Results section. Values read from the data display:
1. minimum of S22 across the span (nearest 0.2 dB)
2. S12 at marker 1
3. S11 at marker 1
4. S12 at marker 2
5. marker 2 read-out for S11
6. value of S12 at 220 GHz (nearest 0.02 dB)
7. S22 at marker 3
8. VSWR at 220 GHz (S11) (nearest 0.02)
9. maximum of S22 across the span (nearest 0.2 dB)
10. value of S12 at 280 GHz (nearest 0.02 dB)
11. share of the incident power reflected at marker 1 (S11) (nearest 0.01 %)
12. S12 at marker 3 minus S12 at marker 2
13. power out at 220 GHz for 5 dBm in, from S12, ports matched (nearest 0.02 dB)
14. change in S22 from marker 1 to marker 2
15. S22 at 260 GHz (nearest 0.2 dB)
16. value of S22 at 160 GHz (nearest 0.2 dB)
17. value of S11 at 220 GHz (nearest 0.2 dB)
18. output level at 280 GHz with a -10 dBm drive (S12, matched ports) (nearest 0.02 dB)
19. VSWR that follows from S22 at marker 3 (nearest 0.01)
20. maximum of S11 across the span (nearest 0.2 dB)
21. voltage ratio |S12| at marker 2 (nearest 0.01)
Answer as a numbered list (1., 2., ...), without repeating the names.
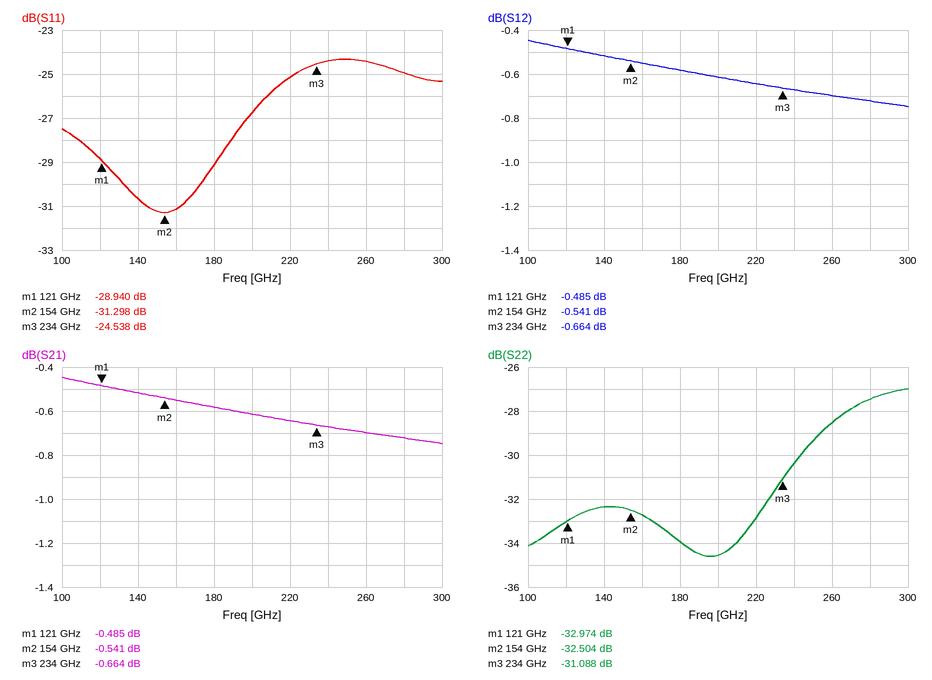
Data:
1. -34.6 dB
2. -0.485 dB
3. -28.940 dB
4. -0.541 dB
5. -31.298 dB
6. -0.64 dB
7. -31.088 dB
8. 1.12
9. -27.0 dB
10. -0.72 dB
11. 0.13 %
12. -0.123 dB
13. 4.36 dBm
14. 0.470 dB
15. -28.6 dB
16. -32.8 dB
17. -25.2 dB
18. -10.72 dBm
19. 1.06
20. -24.4 dB
21. 0.94
